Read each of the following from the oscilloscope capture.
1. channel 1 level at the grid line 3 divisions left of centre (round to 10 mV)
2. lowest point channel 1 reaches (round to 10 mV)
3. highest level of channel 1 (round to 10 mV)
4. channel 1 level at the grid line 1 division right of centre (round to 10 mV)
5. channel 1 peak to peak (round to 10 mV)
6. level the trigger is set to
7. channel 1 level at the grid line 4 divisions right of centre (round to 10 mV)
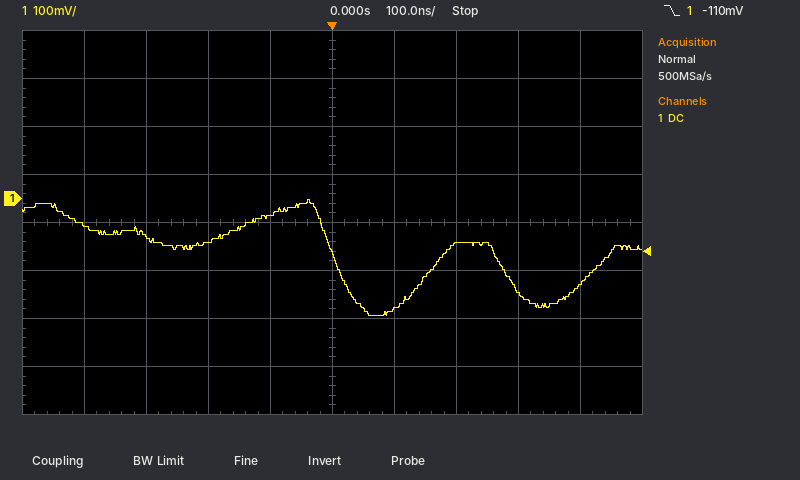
-80 mV
-240 mV
0 mV
-230 mV
240 mV
-110 mV
-180 mV
